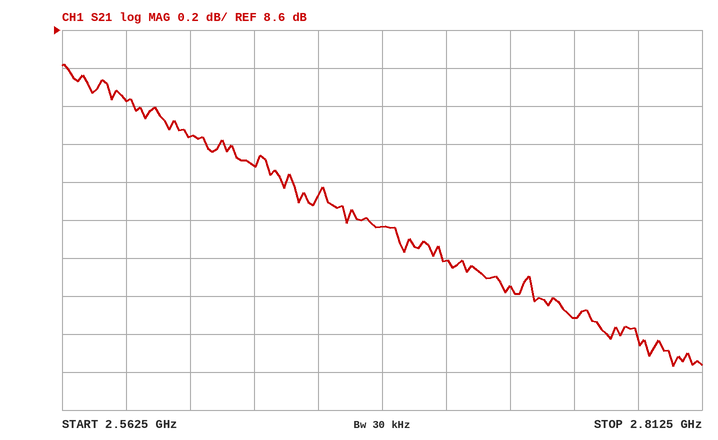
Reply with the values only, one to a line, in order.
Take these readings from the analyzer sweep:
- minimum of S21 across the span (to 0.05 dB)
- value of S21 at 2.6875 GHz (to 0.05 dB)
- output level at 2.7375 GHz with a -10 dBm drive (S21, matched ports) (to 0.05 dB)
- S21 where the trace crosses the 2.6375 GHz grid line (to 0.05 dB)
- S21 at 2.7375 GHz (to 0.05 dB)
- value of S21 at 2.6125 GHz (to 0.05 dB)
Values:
6.85 dB
7.55 dB
-2.75 dBm
7.90 dB
7.25 dB
8.05 dB
